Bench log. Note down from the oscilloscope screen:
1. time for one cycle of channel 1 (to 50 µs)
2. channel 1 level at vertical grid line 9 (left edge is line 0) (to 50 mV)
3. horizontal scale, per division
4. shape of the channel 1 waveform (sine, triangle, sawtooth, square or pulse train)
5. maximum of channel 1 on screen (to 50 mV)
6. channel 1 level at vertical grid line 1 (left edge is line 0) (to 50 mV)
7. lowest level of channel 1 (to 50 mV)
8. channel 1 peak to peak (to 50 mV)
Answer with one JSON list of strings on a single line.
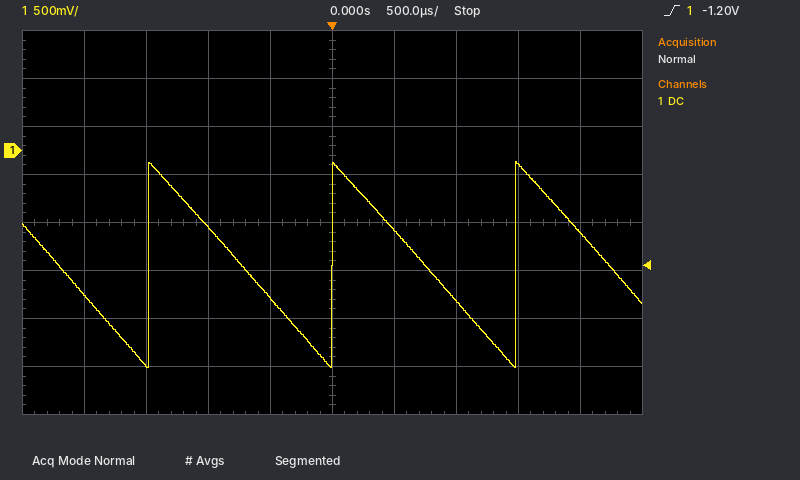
["1.50 ms", "-850 mV", "500 µs", "sawtooth", "-100 mV", "-1.50 V", "-2.25 V", "2.15 V"]
